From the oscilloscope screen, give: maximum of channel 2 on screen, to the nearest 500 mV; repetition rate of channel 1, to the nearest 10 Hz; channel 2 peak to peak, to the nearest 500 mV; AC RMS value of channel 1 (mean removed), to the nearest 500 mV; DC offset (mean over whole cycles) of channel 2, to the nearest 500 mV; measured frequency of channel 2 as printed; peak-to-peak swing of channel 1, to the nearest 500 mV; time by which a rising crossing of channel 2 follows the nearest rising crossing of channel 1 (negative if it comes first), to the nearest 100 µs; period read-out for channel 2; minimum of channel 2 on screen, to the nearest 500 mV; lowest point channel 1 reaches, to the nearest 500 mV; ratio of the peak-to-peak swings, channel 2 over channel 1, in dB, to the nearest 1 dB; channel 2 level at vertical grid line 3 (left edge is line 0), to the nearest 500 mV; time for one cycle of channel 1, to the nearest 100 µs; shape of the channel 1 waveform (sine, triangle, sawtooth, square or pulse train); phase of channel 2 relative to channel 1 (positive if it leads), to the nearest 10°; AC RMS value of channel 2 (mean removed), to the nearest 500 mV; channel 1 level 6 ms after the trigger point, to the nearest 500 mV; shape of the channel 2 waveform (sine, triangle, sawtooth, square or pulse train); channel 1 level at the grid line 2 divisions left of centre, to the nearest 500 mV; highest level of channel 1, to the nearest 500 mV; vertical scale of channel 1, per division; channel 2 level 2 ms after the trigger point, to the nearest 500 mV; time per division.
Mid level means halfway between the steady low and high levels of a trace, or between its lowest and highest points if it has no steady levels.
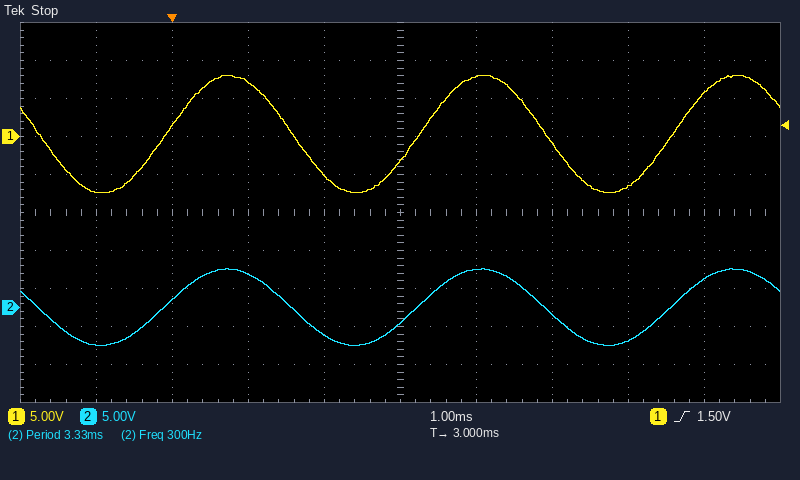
5.0 V
300 Hz
10.0 V
5.5 V
0.0 V
300 Hz
15.5 V
0.0 ms
3.33 ms
-5.0 V
-7.5 V
-4 dB
4.5 V
3.3 ms
sine
0°
3.5 V
-6.5 V
sine
7.0 V
8.0 V
5 V
-3.5 V
1 ms
